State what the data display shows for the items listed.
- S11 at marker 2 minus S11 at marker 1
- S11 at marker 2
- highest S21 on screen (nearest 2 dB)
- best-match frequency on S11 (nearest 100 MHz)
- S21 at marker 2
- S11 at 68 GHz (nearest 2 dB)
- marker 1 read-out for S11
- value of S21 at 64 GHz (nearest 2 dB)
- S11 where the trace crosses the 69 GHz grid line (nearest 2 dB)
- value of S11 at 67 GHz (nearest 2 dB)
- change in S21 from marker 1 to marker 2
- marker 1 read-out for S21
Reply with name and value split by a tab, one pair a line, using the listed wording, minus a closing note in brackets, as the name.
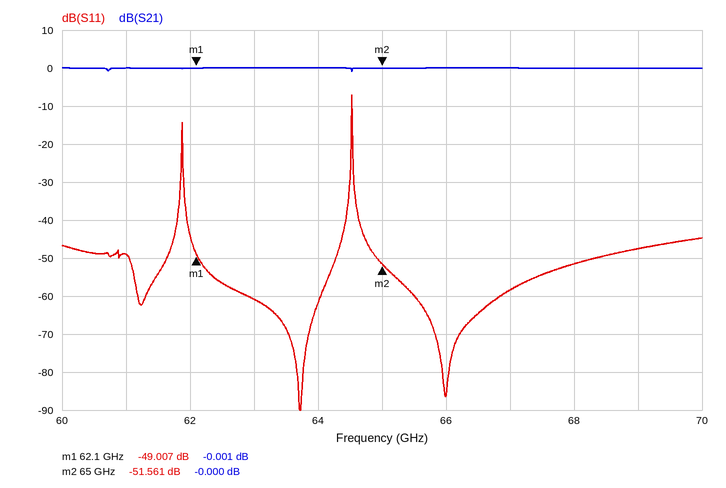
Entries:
S11 at marker 2 minus S11 at marker 1	-2.554 dB
S11 at marker 2	-51.561 dB
highest S21 on screen	0 dB
best-match frequency on S11	63.7 GHz
S21 at marker 2	-0.000 dB
S11 at 68 GHz	-52 dB
marker 1 read-out for S11	-49.007 dB
value of S21 at 64 GHz	0 dB
S11 where the trace crosses the 69 GHz grid line	-48 dB
value of S11 at 67 GHz	-58 dB
change in S21 from marker 1 to marker 2	0.001 dB
marker 1 read-out for S21	-0.001 dB
